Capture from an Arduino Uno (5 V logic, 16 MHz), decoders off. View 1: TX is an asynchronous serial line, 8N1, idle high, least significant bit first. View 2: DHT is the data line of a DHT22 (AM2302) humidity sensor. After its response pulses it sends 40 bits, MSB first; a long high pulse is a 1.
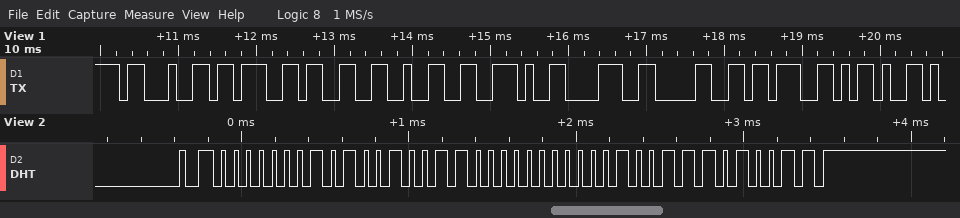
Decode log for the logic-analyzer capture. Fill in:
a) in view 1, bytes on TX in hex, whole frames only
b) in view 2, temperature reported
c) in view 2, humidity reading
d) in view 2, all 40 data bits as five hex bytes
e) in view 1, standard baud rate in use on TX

0x23 0x3B 0x33 0x32 0x2E 0x38 0x30 0x3B 0x2D
-0.9 °C
32.9 %
01 49 80 09 D3
9600 baud
